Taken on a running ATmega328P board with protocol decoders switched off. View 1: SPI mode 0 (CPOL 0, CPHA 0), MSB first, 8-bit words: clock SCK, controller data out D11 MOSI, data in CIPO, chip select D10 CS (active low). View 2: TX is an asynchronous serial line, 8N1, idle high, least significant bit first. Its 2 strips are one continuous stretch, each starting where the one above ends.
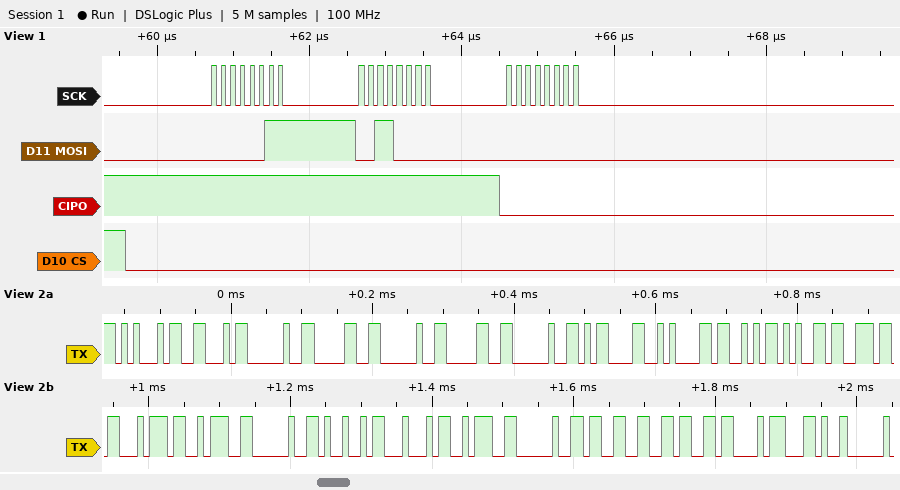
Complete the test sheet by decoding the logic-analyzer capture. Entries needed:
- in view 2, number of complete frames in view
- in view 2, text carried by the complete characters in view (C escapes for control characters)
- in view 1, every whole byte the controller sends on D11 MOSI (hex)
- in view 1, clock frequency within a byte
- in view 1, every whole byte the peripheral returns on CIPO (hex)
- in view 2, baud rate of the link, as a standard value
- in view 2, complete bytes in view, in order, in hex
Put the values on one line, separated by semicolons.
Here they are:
23; "EF 0 0 \r\nSent: ID: 36C,"; 03 30 00; 8 MHz; FF FF 00; 115200 baud; 0x45 0x46 0x20 0x30 0x20 0x30 0x20 0x0D 0x0A 0x53 0x65 0x6E 0x74 0x3A 0x20 0x49 0x44 0x3A 0x20 0x33 0x36 0x43 0x2C
